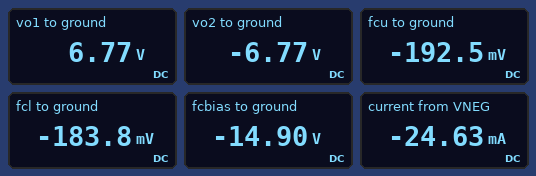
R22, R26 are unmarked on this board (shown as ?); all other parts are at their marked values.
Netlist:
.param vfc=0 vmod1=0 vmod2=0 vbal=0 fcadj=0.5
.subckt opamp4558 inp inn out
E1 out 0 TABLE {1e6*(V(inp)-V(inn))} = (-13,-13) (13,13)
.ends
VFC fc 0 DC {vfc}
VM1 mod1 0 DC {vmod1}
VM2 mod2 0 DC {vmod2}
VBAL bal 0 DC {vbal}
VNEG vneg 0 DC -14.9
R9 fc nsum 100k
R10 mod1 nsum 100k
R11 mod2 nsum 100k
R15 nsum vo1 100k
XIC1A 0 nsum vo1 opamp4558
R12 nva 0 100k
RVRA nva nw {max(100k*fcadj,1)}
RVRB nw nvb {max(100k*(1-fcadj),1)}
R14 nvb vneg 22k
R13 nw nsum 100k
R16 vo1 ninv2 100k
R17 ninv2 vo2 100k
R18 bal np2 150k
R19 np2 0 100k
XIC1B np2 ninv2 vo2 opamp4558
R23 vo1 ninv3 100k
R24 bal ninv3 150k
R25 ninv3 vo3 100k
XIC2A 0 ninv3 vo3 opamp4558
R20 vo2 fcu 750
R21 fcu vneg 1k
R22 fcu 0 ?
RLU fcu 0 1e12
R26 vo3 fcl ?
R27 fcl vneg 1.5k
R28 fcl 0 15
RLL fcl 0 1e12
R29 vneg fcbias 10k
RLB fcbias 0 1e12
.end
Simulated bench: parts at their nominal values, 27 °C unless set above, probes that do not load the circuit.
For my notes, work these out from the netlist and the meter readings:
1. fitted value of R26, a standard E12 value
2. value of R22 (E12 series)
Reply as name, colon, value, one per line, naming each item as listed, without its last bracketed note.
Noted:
fitted value of R26, a standard E12 value: 2.7 kΩ
value of R22: 8.2 Ω
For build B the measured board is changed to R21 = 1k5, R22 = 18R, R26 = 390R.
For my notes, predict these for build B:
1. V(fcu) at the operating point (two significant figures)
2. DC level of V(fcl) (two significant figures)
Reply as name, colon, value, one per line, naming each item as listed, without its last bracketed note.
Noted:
V(fcu) at the operating point: -330 mV
DC level of V(fcl): -390 mV
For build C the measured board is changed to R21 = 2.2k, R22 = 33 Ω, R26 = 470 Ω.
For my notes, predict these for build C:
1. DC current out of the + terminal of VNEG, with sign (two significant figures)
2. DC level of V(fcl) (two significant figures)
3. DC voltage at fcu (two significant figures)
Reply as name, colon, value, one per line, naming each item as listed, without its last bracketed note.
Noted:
DC current out of the + terminal of VNEG, with sign: -16 mA
DC level of V(fcl): -350 mV
DC voltage at fcu: -490 mV
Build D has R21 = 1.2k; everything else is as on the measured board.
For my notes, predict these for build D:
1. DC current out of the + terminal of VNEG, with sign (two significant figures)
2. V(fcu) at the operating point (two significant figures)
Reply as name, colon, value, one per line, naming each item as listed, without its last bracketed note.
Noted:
DC current out of the + terminal of VNEG, with sign: -22 mA
V(fcu) at the operating point: -170 mV
